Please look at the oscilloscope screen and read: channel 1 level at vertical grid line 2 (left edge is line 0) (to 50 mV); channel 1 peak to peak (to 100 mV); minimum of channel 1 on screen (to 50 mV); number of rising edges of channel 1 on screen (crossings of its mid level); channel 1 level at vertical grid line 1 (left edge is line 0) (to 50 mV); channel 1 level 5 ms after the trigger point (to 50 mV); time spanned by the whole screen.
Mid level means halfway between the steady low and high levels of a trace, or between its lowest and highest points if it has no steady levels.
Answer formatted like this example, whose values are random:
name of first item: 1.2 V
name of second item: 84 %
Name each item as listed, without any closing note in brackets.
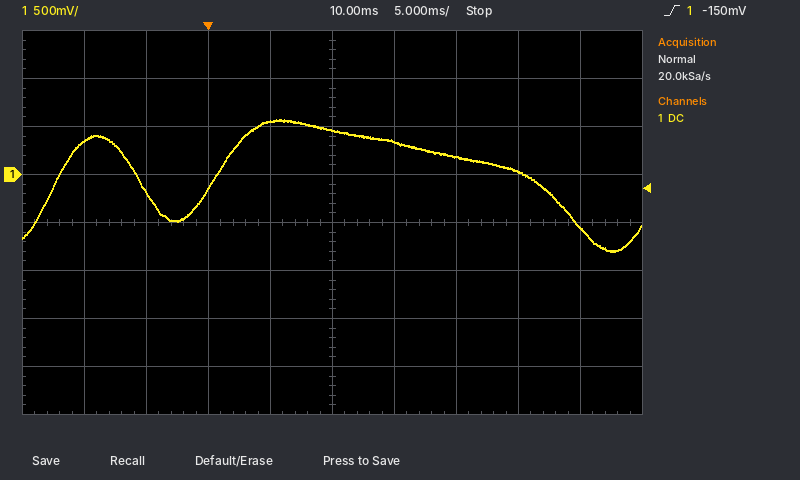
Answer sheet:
channel 1 level at vertical grid line 2 (left edge is line 0): -200 mV
channel 1 peak to peak: 1.40 V
minimum of channel 1 on screen: -800 mV
number of rising edges of channel 1 on screen: 2
channel 1 level at vertical grid line 1 (left edge is line 0): 350 mV
channel 1 level 5 ms after the trigger point: 550 mV
time spanned by the whole screen: 50 ms
